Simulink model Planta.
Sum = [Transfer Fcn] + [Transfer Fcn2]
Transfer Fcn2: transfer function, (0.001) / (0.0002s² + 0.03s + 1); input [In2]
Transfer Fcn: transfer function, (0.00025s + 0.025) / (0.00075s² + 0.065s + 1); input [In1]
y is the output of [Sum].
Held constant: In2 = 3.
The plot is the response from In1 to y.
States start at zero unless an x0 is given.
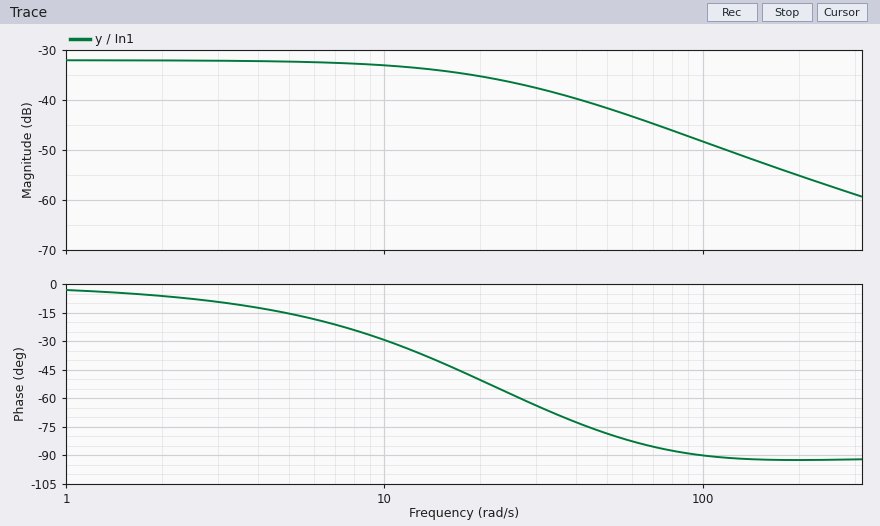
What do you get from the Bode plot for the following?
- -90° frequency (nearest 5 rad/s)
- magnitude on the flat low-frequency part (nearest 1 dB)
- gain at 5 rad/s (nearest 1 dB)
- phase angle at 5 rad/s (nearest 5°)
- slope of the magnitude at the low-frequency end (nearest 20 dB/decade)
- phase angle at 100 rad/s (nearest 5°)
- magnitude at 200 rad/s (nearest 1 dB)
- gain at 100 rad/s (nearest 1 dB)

100 rad/s
-32 dB
-32 dB
-15°
0 dB/decade
-90°
-55 dB
-48 dB
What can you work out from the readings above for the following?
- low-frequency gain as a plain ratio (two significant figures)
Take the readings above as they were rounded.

0.025
